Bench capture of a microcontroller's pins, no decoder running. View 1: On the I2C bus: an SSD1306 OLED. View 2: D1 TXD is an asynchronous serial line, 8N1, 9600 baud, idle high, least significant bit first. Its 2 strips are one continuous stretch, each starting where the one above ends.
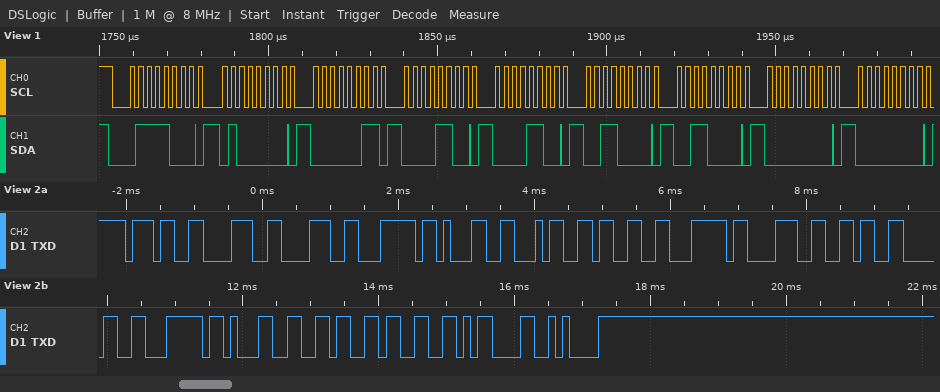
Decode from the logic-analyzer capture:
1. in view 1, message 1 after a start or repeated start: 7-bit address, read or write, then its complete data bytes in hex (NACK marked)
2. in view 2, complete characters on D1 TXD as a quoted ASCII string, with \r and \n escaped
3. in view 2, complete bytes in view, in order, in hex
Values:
0x3C write: 40 03 0C 0C 30 30 00 00
"788|143|860|163\r\n"
37 38 38 7C 31 34 33 7C 38 36 30 7C 31 36 33 0D 0A
